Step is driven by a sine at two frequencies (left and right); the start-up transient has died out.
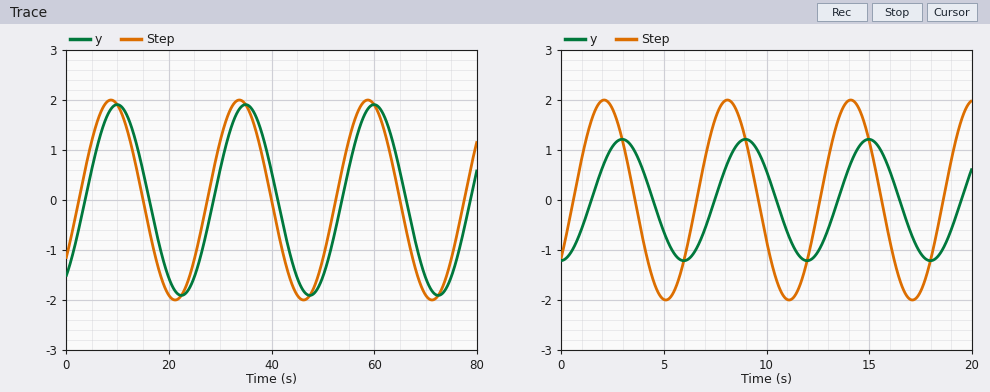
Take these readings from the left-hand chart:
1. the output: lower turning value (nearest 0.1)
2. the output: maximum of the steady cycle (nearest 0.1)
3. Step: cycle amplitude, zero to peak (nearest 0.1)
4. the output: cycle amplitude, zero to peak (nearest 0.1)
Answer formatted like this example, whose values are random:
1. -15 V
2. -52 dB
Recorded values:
1. -1.9
2. 1.9
3. 2.0
4. 1.9
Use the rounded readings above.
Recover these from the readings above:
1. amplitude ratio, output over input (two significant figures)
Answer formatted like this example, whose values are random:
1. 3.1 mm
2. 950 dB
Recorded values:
1. 0.95
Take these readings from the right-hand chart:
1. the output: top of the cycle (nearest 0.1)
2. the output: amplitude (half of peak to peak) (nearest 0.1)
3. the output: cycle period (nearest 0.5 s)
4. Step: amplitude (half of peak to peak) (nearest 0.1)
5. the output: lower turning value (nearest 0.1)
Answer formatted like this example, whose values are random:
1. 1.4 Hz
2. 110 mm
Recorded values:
1. 1.2
2. 1.2
3. 6.0 s
4. 2.0
5. -1.2
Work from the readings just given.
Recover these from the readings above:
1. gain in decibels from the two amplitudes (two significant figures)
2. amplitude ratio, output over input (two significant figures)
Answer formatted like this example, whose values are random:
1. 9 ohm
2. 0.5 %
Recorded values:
1. -4.4 dB
2. 0.60
